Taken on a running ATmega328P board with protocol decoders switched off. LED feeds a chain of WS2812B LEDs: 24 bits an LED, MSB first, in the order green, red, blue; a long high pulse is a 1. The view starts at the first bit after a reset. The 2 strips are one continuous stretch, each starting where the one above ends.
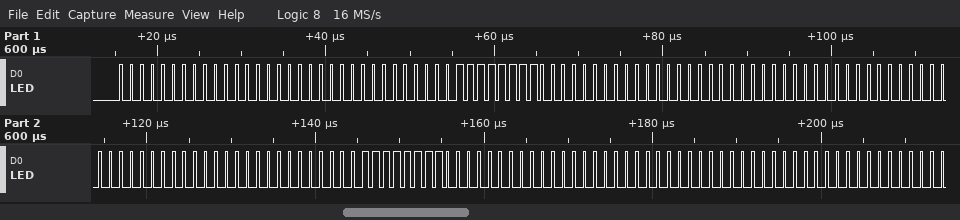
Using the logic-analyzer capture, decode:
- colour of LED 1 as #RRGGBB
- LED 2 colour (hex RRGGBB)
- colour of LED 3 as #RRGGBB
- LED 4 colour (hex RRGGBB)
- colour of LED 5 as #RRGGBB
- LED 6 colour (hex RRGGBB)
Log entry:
#000000
#FF0000
#000000
#000000
#FF0000
#000000
